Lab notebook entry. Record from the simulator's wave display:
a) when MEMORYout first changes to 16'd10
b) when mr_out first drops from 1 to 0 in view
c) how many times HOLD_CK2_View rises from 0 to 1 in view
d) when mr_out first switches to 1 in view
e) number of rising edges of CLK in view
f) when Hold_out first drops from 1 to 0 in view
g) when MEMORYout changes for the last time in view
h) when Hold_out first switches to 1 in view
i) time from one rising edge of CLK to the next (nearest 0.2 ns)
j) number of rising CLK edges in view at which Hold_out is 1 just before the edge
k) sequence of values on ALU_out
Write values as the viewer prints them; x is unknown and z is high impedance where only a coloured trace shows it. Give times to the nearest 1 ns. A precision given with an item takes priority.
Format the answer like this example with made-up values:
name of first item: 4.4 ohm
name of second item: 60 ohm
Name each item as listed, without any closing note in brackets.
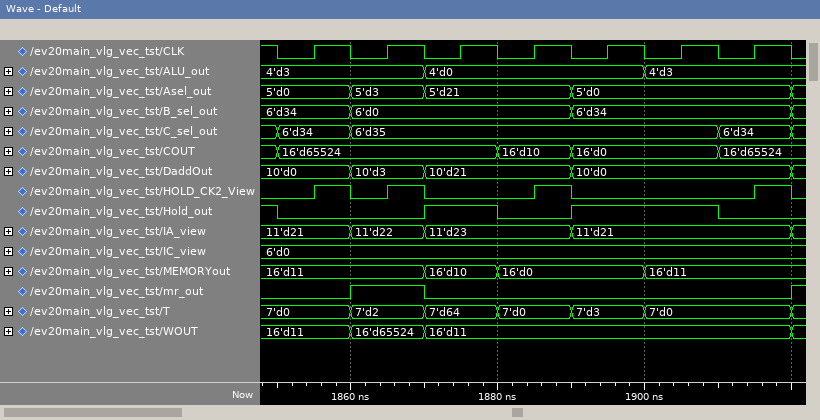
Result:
when MEMORYout first changes to 16'd10: 1870 ns
when mr_out first drops from 1 to 0 in view: 1870 ns
how many times HOLD_CK2_View rises from 0 to 1 in view: 4
when mr_out first switches to 1 in view: 1860 ns
number of rising edges of CLK in view: 7
when Hold_out first drops from 1 to 0 in view: 1850 ns
when MEMORYout changes for the last time in view: 1900 ns
when Hold_out first switches to 1 in view: 1870 ns
time from one rising edge of CLK to the next: 10 ns
number of rising CLK edges in view at which Hold_out is 1 just before the edge: 3
sequence of values on ALU_out: 4'd3, 4'd0, 4'd3
